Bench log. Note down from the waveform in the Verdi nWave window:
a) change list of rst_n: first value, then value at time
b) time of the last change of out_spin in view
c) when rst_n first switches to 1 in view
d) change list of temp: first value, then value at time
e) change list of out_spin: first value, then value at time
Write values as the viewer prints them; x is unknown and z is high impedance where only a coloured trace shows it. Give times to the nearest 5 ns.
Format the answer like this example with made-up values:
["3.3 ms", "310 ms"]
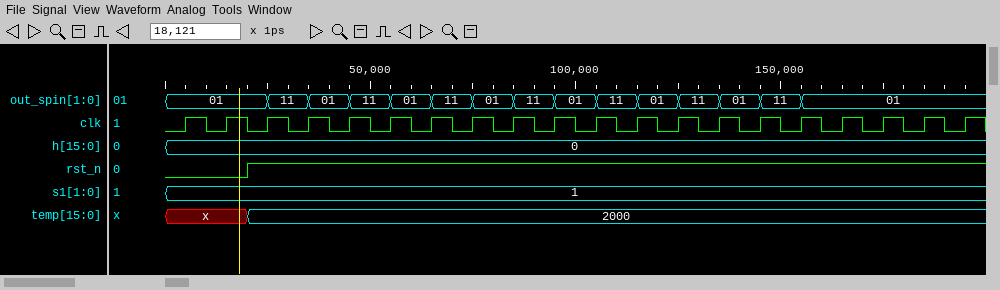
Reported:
["0, 1 at 20 ns", "155 ns", "20 ns", "x, 2000 at 20 ns", "01, 11 at 25 ns, 01 at 35 ns, 11 at 45 ns, 01 at 55 ns, 11 at 65 ns, 01 at 75 ns, 11 at 85 ns, 01 at 95 ns, 11 at 105 ns, 01 at 115 ns, 11 at 125 ns, 01 at 135 ns, 11 at 145 ns, 01 at 155 ns"]
